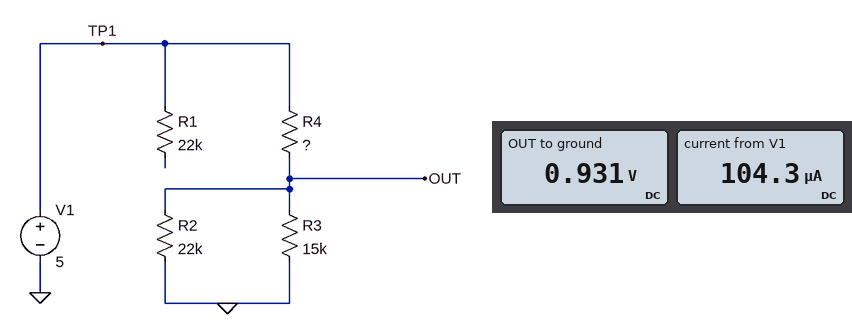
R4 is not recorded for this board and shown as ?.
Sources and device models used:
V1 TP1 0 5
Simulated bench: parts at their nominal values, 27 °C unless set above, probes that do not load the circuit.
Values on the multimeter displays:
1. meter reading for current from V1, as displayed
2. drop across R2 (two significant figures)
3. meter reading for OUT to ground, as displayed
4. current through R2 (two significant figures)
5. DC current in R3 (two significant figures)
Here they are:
104.3 µA
930 mV
0.931 V
42 µA
62 µA
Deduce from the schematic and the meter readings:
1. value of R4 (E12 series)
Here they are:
39 kΩ
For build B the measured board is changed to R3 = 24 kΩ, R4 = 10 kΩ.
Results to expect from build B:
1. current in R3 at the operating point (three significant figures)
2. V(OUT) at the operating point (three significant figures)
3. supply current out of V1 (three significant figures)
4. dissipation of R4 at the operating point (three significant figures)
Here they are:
111 µA
2.67 V
233 µA
542 µW
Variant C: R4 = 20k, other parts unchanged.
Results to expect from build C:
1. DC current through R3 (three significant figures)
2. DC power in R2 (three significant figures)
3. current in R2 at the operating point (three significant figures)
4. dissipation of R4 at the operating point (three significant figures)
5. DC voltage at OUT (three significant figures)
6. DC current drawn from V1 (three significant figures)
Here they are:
103 µA
108 µW
70.1 µA
598 µW
1.54 V
173 µA
